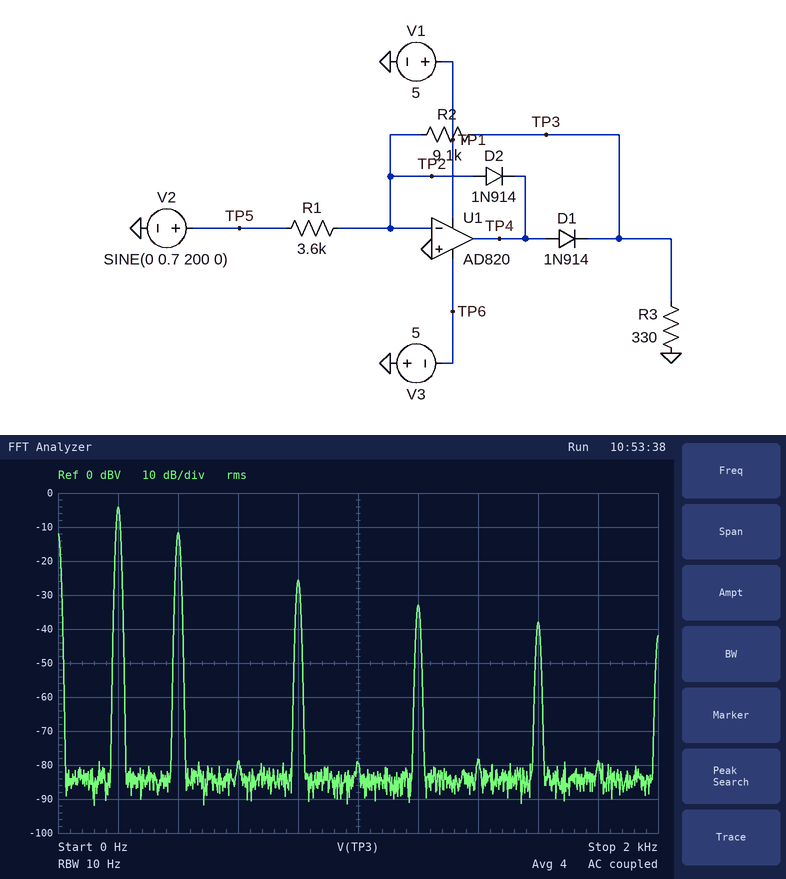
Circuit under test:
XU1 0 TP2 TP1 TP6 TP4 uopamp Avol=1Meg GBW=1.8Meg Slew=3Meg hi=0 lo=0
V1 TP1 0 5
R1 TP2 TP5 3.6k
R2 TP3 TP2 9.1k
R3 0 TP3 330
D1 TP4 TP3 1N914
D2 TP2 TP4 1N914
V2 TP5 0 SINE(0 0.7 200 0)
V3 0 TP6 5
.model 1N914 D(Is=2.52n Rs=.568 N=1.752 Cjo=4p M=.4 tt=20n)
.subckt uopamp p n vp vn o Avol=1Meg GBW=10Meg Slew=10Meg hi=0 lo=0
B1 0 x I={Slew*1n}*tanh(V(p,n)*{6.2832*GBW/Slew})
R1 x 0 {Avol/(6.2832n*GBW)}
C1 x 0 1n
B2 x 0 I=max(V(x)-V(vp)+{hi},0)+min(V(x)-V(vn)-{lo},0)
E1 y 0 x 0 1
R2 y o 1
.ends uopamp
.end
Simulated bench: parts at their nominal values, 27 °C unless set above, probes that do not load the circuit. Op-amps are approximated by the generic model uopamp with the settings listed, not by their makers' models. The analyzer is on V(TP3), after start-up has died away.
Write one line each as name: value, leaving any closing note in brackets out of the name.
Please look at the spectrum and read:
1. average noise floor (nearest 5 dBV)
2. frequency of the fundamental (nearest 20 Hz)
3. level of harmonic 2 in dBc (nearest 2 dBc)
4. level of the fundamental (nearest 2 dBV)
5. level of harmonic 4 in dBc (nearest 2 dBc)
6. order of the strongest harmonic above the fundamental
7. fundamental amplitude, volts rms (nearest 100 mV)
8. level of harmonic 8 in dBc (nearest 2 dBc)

average noise floor: -85 dBV
frequency of the fundamental: 200 Hz
level of harmonic 2 in dBc: -8 dBc
level of the fundamental: -4 dBV
level of harmonic 4 in dBc: -22 dBc
order of the strongest harmonic above the fundamental: 2
fundamental amplitude, volts rms: 600 mV
level of harmonic 8 in dBc: -34 dBc
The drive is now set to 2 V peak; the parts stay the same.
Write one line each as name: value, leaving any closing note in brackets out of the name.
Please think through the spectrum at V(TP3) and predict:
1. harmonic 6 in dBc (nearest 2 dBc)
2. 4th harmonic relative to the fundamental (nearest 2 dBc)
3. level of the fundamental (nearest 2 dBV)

harmonic 6 in dBc: -34 dBc
4th harmonic relative to the fundamental: -18 dBc
level of the fundamental: 4 dBV
